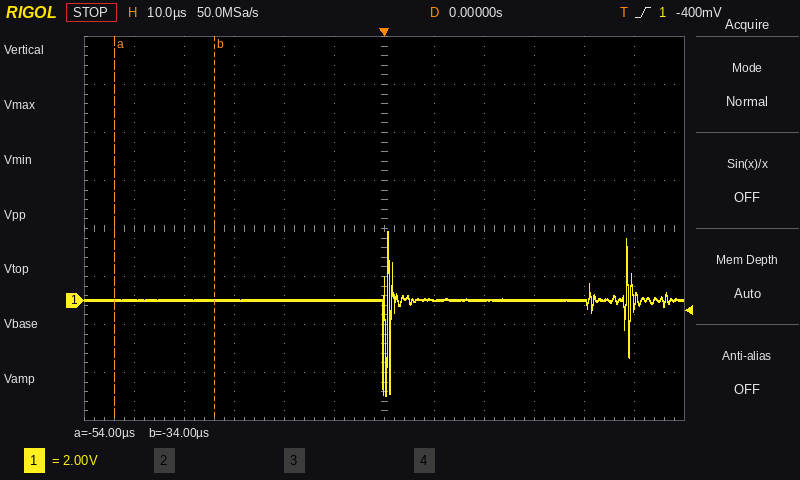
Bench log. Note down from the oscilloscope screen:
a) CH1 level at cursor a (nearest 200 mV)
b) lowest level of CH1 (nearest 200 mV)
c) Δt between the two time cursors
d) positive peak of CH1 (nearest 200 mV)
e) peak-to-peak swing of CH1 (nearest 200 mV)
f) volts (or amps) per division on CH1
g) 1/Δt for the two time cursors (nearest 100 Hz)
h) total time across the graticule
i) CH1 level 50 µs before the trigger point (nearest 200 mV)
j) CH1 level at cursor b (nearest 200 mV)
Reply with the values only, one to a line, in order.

0.0 V
-4.0 V
20 µs
2.8 V
6.8 V
2 V
50.0 kHz
120 µs
0.0 V
0.0 V
